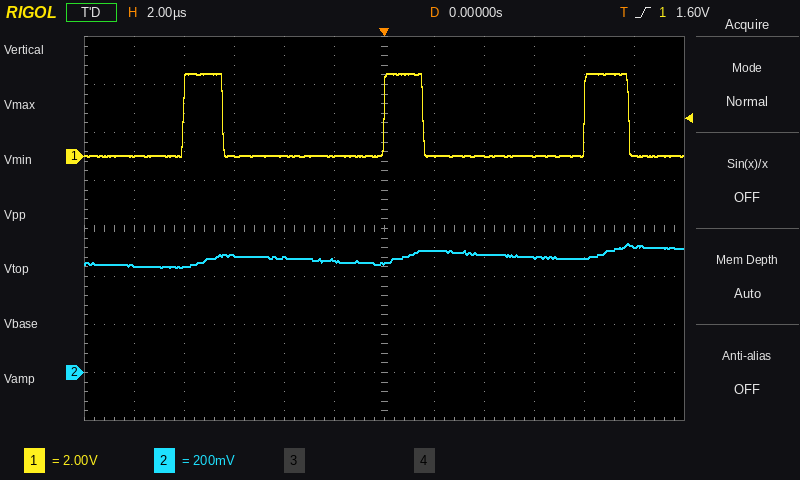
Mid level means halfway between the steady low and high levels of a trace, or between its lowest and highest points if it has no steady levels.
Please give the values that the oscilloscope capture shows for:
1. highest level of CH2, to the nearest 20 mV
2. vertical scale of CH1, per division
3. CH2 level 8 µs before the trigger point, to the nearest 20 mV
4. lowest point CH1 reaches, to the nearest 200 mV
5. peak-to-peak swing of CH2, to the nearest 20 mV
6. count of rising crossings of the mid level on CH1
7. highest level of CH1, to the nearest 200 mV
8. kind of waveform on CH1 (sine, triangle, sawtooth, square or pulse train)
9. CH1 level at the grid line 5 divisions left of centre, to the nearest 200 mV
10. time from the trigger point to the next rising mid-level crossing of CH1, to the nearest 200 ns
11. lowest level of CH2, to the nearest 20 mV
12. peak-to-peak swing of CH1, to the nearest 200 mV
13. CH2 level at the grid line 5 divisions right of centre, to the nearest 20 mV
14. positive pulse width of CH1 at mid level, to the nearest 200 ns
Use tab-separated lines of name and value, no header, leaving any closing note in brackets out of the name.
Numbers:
highest level of CH2, to the nearest 20 mV	540 mV
vertical scale of CH1, per division	2 V
CH2 level 8 µs before the trigger point, to the nearest 20 mV	440 mV
lowest point CH1 reaches, to the nearest 200 mV	0.0 V
peak-to-peak swing of CH2, to the nearest 20 mV	100 mV
count of rising crossings of the mid level on CH1	3
highest level of CH1, to the nearest 200 mV	3.4 V
kind of waveform on CH1	pulse train
CH1 level at the grid line 5 divisions left of centre, to the nearest 200 mV	0.0 V
time from the trigger point to the next rising mid-level crossing of CH1, to the nearest 200 ns	8.0 µs
lowest level of CH2, to the nearest 20 mV	440 mV
peak-to-peak swing of CH1, to the nearest 200 mV	3.4 V
CH2 level at the grid line 5 divisions right of centre, to the nearest 20 mV	520 mV
positive pulse width of CH1 at mid level, to the nearest 200 ns	1.6 µs
